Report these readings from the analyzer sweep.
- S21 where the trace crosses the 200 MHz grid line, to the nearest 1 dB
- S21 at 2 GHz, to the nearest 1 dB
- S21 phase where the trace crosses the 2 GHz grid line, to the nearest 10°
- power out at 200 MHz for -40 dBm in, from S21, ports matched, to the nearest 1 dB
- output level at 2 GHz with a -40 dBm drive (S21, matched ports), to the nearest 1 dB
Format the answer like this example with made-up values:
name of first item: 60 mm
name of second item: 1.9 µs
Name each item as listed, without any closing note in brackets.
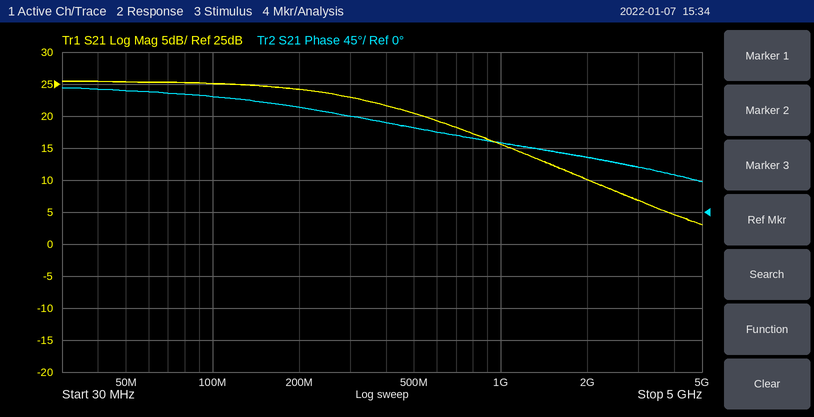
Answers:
S21 where the trace crosses the 200 MHz grid line, to the nearest 1 dB: 24 dB
S21 at 2 GHz, to the nearest 1 dB: 10 dB
S21 phase where the trace crosses the 2 GHz grid line, to the nearest 10°: 80°
power out at 200 MHz for -40 dBm in, from S21, ports matched, to the nearest 1 dB: -16 dBm
output level at 2 GHz with a -40 dBm drive (S21, matched ports), to the nearest 1 dB: -30 dBm
